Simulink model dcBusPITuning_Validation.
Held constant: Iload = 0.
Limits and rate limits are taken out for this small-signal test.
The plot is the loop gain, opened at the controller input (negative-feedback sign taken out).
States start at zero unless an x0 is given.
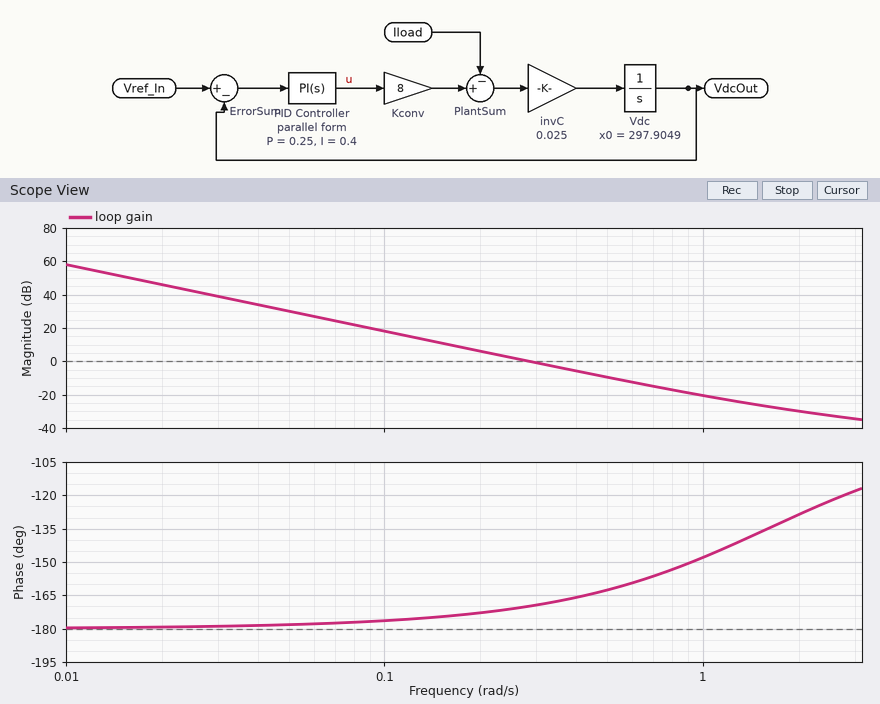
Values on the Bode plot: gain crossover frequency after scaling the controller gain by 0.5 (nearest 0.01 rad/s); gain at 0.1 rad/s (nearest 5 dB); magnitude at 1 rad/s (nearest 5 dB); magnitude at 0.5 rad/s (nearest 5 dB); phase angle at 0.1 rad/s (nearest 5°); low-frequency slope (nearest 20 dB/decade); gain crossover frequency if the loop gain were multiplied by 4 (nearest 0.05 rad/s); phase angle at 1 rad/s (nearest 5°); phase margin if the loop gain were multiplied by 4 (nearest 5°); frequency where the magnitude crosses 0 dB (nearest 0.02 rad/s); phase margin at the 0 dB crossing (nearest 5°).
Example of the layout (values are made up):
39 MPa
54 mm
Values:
0.20 rad/s
20 dB
-20 dB
-10 dB
-175°
-40 dB/decade
0.60 rad/s
-150°
20°
0.28 rad/s
10°
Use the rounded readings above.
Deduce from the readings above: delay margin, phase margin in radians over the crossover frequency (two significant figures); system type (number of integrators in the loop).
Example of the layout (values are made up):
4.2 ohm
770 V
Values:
0.62 s
2
